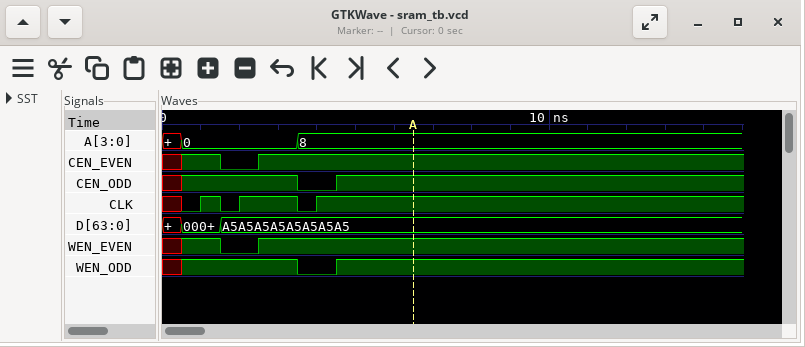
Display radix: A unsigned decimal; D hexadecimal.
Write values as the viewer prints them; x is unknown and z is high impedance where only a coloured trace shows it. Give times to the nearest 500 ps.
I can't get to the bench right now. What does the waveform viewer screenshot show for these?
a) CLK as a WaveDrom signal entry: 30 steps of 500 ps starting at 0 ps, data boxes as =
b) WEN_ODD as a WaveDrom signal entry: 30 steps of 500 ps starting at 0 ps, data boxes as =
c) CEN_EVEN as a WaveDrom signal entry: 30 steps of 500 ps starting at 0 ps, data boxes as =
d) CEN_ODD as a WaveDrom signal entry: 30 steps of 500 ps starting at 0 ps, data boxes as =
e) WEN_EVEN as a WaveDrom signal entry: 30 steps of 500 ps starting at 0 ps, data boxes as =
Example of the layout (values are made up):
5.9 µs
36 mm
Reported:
{name: 'CLK', wave: 'x0101..01.....................'}
{name: 'WEN_ODD', wave: 'x1.....0.1....................'}
{name: 'CEN_EVEN', wave: 'x1.0.1........................'}
{name: 'CEN_ODD', wave: 'x1.....0.1....................'}
{name: 'WEN_EVEN', wave: 'x1.0.1........................'}
